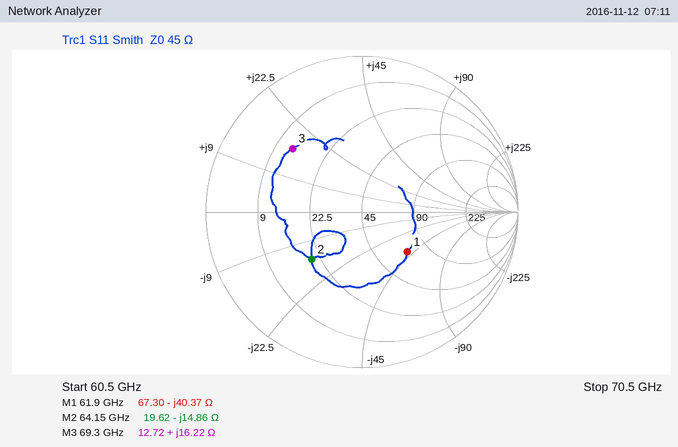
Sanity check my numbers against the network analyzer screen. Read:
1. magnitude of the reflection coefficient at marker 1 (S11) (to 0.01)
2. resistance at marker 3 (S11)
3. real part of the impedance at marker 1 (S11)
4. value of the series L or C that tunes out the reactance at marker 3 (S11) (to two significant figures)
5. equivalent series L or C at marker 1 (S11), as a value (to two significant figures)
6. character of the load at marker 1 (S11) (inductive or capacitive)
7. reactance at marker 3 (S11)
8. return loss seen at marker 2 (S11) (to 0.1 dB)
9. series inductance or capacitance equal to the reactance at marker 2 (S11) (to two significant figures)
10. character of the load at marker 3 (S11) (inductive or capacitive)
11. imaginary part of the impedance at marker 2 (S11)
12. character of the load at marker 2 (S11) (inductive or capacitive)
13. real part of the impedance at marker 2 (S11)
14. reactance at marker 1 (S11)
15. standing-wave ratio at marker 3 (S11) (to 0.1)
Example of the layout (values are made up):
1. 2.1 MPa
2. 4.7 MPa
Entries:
1. 0.39
2. 12.72 Ω
3. 67.30 Ω
4. 140 fF
5. 64 fF
6. capacitive
7. +16.22 Ω
8. 7.1 dB
9. 170 fF
10. inductive
11. -14.86 Ω
12. capacitive
13. 19.62 Ω
14. -40.37 Ω
15. 4.0
